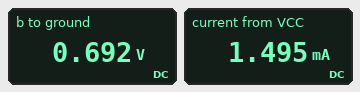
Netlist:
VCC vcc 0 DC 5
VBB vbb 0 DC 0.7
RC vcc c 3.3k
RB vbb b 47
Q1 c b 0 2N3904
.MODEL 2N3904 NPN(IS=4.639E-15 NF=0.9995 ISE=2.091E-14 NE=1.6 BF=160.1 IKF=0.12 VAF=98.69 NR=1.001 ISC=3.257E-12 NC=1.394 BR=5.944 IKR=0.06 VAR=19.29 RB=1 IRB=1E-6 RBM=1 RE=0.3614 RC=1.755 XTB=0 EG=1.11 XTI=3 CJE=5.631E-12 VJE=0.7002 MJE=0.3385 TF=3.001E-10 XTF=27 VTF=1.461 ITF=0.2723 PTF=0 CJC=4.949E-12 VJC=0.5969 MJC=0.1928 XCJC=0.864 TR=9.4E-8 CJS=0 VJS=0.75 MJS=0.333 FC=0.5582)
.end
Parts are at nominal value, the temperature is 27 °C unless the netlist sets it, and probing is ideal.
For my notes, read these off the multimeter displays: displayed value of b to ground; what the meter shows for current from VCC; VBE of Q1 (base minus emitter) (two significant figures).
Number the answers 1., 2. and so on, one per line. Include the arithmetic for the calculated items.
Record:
1. 0.692 V
2. 1.495 mA
3. 692 mV = 690 mV
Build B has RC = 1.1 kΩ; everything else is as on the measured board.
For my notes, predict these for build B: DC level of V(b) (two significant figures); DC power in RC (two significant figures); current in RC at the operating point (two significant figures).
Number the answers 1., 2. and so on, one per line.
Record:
1. 700 mV
2. 6.4 mW
3. 2.4 mA
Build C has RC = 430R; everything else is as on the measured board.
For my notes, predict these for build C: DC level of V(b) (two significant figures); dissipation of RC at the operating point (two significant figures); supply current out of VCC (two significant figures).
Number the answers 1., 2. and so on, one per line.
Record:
1. 700 mV
2. 2.6 mW
3. 2.4 mA
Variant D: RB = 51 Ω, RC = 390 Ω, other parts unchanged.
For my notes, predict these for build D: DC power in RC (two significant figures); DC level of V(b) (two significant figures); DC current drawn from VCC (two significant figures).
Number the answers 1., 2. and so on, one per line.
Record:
1. 2.3 mW
2. 700 mV
3. 2.4 mA
